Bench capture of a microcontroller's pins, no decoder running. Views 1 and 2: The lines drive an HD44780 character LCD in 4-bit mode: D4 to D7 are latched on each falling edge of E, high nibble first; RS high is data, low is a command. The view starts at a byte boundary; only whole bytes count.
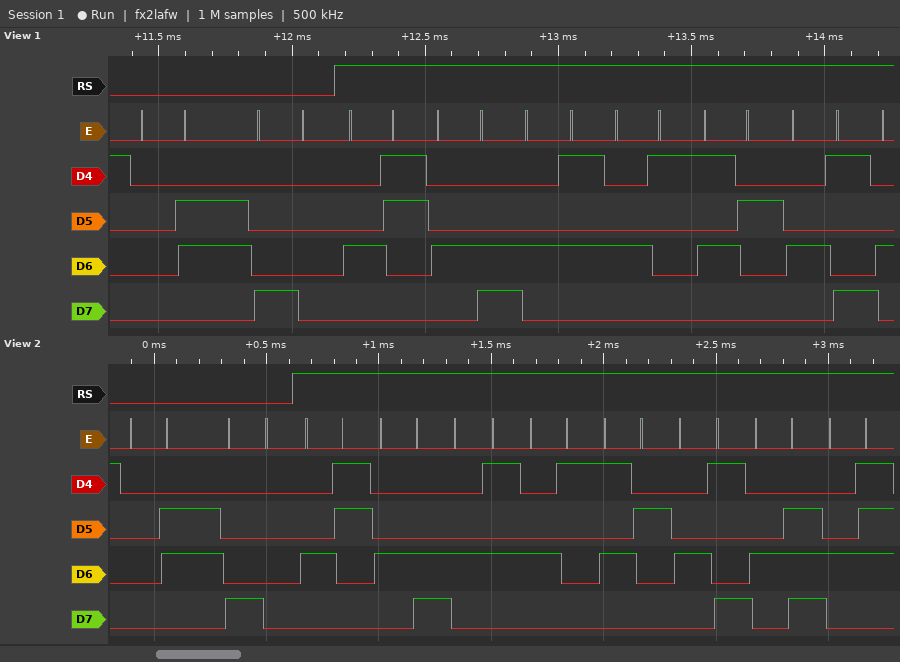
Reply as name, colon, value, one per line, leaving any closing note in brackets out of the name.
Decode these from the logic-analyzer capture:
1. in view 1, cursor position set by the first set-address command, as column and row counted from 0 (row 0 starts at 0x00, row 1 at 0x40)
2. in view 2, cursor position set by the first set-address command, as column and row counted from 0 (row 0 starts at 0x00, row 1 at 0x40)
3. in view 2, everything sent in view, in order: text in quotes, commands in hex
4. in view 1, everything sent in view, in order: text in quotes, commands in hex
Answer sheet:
in view 1, cursor position set by the first set-address command, as column and row counted from 0: column 0, row 0
in view 2, cursor position set by the first set-address command, as column and row counted from 0: column 0, row 0
in view 2, everything sent in view, in order: text in quotes, commands in hex: 0x06 0x80 "CLEARING"
in view 1, everything sent in view, in order: text in quotes, commands in hex: 0x06 0x80 "CLEARI"
